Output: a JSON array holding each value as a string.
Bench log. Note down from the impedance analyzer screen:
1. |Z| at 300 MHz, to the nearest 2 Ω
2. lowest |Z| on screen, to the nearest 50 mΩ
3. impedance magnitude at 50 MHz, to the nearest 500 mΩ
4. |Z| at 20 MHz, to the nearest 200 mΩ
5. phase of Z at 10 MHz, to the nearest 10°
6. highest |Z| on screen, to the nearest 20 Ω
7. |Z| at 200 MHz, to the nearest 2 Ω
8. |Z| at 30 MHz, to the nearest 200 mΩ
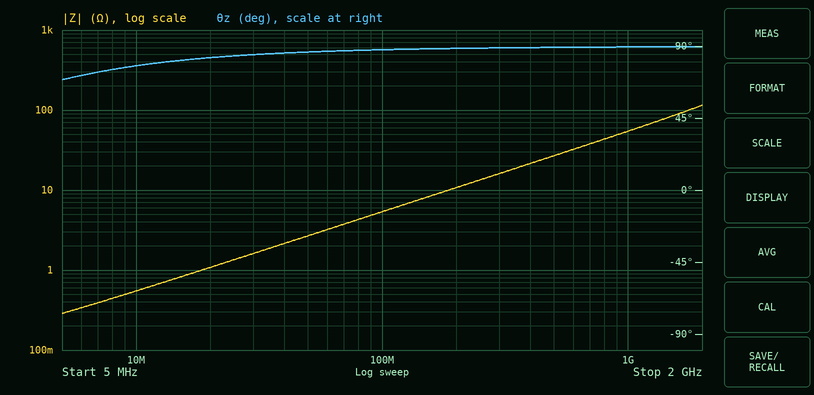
["16 Ω", "300 mΩ", "2.5 Ω", "1.0 Ω", "80°", "120 Ω", "10 Ω", "1.6 Ω"]
